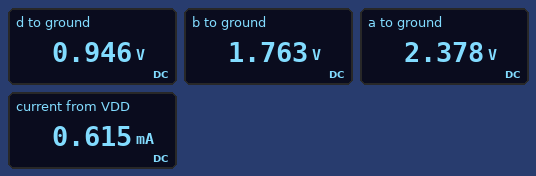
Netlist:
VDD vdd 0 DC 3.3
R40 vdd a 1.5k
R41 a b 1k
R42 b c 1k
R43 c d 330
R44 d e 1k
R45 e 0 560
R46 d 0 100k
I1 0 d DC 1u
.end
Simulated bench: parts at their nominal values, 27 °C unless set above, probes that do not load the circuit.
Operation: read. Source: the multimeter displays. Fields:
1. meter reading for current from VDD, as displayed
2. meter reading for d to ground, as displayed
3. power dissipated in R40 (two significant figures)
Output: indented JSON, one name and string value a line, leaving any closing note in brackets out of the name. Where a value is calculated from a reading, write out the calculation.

{
  "meter reading for current from VDD, as displayed": "0.615 mA",
  "meter reading for d to ground, as displayed": "0.946 V",
  "power dissipated in R40": "(3.3 V - 2.378 V)^2 / 1.5 kΩ = 570 µW"
}
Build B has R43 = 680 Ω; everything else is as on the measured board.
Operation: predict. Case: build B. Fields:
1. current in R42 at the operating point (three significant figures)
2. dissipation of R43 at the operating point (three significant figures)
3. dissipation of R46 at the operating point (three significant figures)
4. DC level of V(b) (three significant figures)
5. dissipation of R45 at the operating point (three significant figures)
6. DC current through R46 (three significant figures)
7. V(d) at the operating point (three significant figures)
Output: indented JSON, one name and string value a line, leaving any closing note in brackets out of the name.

{
  "current in R42 at the operating point": "577 µA",
  "dissipation of R43 at the operating point": "226 µW",
  "dissipation of R46 at the operating point": "7.88 µW",
  "DC level of V(b)": "1.86 V",
  "dissipation of R45 at the operating point": "181 µW",
  "DC current through R46": "8.88 µA",
  "V(d) at the operating point": "888 mV"
}
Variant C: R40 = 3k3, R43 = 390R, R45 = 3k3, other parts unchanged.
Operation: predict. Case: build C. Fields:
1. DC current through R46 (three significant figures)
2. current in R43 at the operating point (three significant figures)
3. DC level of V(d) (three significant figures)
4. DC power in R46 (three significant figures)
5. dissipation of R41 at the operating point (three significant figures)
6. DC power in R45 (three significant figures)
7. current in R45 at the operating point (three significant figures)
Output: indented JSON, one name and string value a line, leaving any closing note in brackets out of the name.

{
  "DC current through R46": "13.9 µA",
  "current in R43 at the operating point": "336 µA",
  "DC level of V(d)": "1.39 V",
  "DC power in R46": "19.3 µW",
  "dissipation of R41 at the operating point": "113 µW",
  "DC power in R45": "344 µW",
  "current in R45 at the operating point": "323 µA"
}
